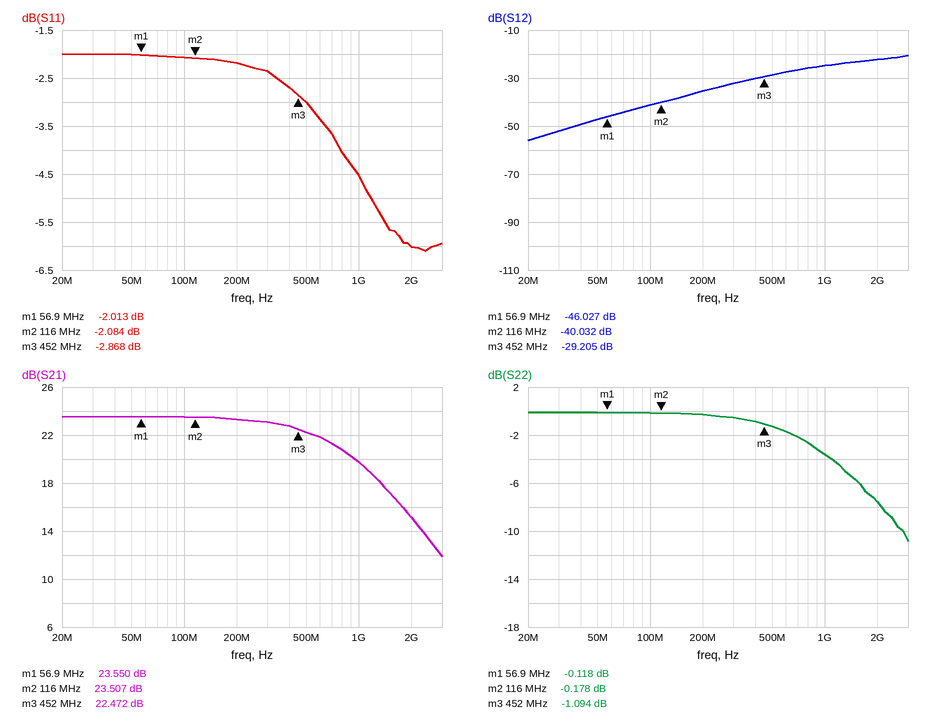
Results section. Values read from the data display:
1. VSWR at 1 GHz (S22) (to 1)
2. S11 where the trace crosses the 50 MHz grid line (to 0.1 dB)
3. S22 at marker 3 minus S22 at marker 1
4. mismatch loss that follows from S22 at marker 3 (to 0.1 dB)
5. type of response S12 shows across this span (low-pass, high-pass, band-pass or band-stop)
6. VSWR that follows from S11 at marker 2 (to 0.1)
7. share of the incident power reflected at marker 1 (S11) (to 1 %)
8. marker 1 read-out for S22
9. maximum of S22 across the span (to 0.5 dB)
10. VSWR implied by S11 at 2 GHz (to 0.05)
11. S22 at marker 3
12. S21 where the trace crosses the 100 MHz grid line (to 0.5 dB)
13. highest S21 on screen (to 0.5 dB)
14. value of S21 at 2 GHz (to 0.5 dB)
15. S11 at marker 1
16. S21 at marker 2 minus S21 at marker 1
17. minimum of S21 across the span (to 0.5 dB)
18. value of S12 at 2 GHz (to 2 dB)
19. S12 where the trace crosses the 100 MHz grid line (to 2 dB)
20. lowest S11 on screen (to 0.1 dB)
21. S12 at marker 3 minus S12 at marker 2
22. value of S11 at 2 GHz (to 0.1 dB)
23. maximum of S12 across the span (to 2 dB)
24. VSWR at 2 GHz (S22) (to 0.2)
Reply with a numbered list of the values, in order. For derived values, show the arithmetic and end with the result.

1. |Γ| = 10^(-3.5/20) = 0.6683; VSWR = (1 + 0.6683)/(1 − 0.6683) ≈ 5
2. -2.0 dB
3. -1.094 − (-0.118) = -0.976 dB
4. −10 log10(1 − 10^(-1.094/10)) ≈ 6.5 dB
5. high-pass
6. (1 + 0.7867)/(1 − 0.7867) ≈ 8.4
7. 10^(-2.013/10) ≈ 63 %
8. -0.118 dB
9. 0.0 dB
10. |Γ| = 10^(-6/20) = 0.5012; VSWR = (1 + 0.5012)/(1 − 0.5012) ≈ 3.01, so 3.00 to the nearest 0.05
11. -1.094 dB
12. 23.5 dB
13. 23.5 dB
14. 15.0 dB
15. -2.013 dB
16. 23.507 − (23.55) = -0.043 dB
17. 12.0 dB
18. -22 dB
19. -42 dB
20. -6.1 dB
21. -29.205 − (-40.032) = 10.827 dB
22. -6.0 dB
23. -20 dB
24. |Γ| = 10^(-7.5/20) = 0.4217; VSWR = (1 + 0.4217)/(1 − 0.4217) ≈ 2.46, so 2.4 to the nearest 0.2
